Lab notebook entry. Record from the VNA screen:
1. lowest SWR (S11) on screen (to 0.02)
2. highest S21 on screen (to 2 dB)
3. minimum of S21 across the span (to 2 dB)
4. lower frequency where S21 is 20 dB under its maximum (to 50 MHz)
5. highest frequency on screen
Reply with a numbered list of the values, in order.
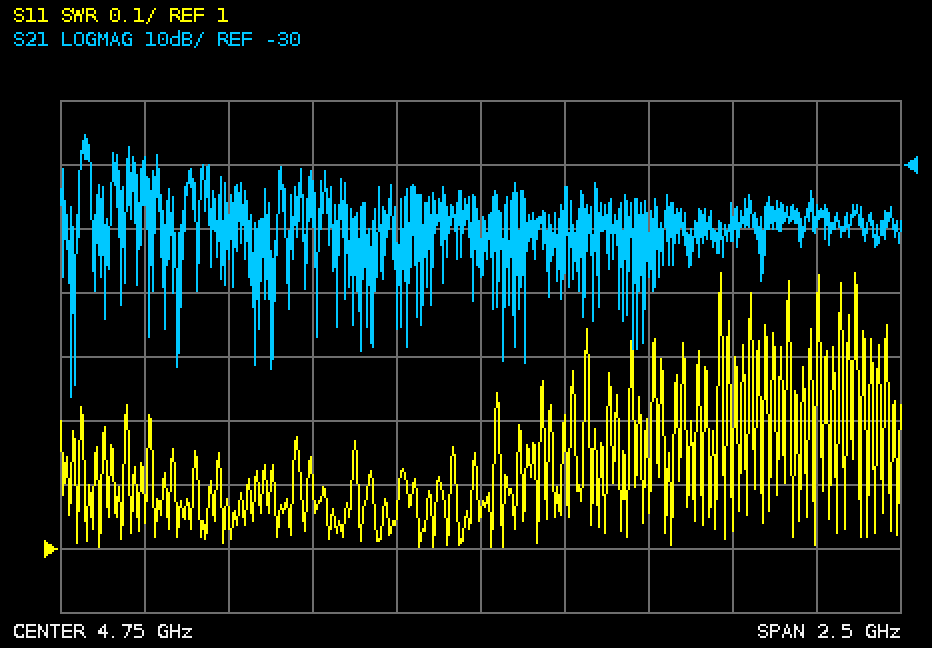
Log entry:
1. 1.00
2. -26 dB
3. -66 dB
4. 3.55 GHz
5. 6 GHz
